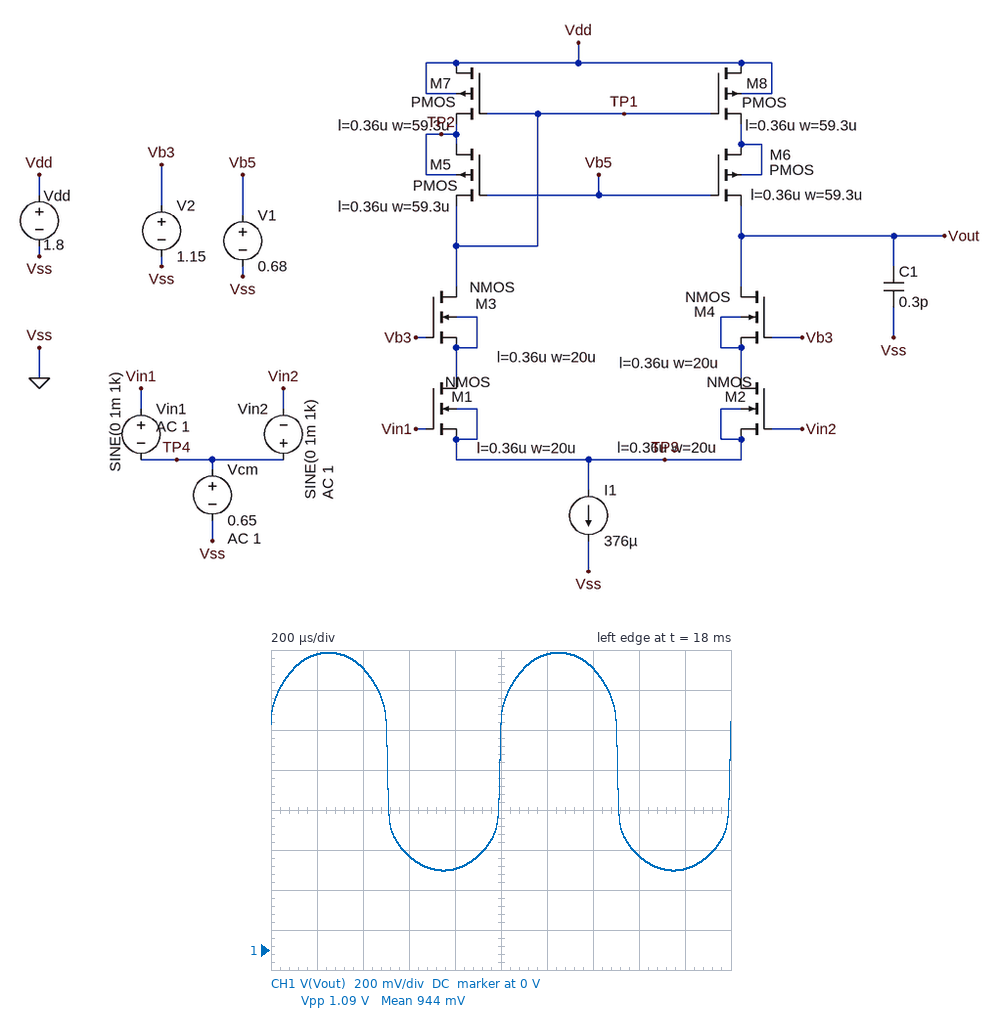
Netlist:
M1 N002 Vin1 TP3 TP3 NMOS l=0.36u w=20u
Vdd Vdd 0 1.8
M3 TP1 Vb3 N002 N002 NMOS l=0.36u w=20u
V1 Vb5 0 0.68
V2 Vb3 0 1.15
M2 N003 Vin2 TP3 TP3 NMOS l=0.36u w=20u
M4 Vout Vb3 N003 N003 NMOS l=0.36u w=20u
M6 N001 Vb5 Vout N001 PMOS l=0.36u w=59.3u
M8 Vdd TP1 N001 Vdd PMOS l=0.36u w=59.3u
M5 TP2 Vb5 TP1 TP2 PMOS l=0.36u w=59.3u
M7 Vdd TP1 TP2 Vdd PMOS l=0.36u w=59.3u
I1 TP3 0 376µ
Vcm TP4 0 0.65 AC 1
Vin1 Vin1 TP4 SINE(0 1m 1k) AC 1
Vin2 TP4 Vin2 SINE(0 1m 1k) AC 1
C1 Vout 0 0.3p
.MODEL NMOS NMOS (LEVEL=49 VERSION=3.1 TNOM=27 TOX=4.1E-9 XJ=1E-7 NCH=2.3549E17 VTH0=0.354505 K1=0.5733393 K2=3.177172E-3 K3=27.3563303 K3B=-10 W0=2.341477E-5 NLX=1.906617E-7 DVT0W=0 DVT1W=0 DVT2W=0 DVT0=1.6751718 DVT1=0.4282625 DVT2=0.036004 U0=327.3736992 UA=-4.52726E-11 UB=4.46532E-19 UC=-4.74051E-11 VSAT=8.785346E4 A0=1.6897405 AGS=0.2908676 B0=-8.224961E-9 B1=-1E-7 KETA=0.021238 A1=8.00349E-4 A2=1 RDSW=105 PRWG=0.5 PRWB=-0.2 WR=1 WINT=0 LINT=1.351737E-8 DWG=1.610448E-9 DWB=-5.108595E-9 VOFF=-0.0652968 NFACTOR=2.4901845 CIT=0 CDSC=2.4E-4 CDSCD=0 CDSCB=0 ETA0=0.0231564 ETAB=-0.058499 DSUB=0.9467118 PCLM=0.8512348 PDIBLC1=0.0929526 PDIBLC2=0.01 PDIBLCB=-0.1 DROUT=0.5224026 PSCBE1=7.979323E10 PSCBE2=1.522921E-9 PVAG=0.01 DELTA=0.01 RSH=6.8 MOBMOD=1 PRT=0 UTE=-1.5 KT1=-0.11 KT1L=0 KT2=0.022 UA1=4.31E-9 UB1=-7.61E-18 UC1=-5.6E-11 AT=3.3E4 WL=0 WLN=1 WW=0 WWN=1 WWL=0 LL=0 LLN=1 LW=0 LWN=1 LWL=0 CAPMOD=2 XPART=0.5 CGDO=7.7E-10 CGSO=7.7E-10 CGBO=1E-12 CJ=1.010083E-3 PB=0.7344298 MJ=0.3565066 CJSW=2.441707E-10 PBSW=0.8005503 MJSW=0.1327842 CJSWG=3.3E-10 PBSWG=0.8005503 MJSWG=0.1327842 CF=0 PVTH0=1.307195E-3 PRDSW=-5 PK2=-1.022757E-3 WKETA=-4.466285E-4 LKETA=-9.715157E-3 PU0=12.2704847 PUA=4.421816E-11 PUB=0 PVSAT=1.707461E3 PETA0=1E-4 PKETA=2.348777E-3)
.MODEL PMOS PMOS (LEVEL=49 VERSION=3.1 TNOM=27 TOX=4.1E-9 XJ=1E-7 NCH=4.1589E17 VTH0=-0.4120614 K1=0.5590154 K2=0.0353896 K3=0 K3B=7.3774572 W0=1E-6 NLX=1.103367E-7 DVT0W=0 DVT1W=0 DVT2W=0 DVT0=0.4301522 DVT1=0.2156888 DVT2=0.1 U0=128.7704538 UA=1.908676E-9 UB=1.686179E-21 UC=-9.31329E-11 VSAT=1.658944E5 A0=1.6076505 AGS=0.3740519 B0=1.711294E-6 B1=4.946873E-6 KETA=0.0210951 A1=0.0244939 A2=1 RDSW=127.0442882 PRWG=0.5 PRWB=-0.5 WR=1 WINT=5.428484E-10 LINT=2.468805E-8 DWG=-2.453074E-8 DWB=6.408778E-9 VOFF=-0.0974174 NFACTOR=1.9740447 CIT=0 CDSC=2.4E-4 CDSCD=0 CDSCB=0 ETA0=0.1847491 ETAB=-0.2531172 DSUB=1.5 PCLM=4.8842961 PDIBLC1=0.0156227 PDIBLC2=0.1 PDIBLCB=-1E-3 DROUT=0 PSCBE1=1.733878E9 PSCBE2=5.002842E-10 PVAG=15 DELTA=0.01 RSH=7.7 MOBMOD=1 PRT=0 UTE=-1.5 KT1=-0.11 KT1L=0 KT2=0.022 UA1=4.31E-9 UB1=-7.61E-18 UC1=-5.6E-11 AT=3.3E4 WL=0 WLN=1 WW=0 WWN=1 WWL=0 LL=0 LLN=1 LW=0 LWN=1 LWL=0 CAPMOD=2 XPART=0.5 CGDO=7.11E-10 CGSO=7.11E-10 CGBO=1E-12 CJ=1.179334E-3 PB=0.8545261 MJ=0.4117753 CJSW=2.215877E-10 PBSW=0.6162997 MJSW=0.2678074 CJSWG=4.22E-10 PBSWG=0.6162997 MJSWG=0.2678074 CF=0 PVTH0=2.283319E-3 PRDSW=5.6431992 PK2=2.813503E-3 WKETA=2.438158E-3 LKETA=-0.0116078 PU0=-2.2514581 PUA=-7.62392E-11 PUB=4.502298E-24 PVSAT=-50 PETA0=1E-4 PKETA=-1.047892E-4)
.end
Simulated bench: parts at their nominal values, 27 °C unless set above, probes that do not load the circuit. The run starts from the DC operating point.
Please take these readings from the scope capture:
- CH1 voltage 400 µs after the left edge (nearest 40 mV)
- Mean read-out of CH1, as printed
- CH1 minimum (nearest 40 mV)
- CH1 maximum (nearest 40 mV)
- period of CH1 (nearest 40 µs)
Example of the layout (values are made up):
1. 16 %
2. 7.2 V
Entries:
1. 1.40 V
2. 944 mV
3. 400 mV
4. 1.48 V
5. 1.00 ms
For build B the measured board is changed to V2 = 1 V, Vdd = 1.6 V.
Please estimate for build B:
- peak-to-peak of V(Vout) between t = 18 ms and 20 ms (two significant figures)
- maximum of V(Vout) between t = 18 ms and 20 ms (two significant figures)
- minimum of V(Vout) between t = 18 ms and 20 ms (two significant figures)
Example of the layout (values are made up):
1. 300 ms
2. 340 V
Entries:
1. 1.0 V
2. 1.3 V
3. 310 mV
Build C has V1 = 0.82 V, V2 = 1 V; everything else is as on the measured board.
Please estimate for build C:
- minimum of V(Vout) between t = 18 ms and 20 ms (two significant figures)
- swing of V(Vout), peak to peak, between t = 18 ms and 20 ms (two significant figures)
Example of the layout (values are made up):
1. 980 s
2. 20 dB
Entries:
1. 310 mV
2. 1.2 V
